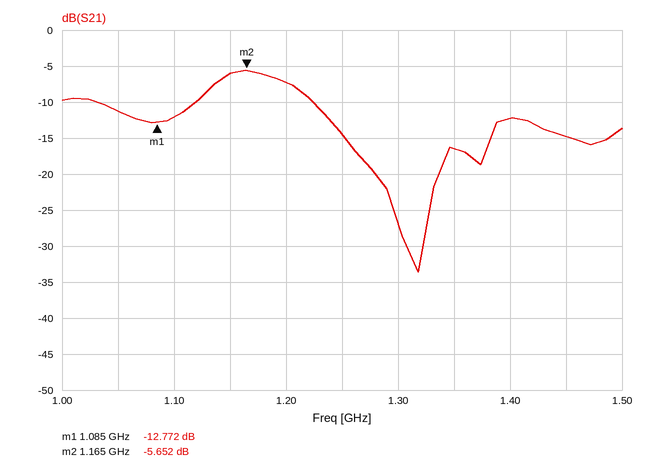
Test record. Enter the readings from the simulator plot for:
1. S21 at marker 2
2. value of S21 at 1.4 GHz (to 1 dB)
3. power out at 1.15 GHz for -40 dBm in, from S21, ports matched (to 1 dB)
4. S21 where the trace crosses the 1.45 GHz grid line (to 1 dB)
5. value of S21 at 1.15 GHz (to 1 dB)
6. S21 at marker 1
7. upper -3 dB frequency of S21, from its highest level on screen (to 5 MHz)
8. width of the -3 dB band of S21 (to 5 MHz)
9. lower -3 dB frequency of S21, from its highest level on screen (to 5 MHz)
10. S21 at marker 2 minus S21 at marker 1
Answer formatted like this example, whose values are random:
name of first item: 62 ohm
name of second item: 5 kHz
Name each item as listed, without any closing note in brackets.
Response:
S21 at marker 2: -5.652 dB
value of S21 at 1.4 GHz: -12 dB
power out at 1.15 GHz for -40 dBm in, from S21, ports matched: -46 dBm
S21 where the trace crosses the 1.45 GHz grid line: -15 dB
value of S21 at 1.15 GHz: -6 dB
S21 at marker 1: -12.772 dB
upper -3 dB frequency of S21, from its highest level on screen: 1.215 GHz
width of the -3 dB band of S21: 85 MHz
lower -3 dB frequency of S21, from its highest level on screen: 1.130 GHz
S21 at marker 2 minus S21 at marker 1: 7.120 dB
